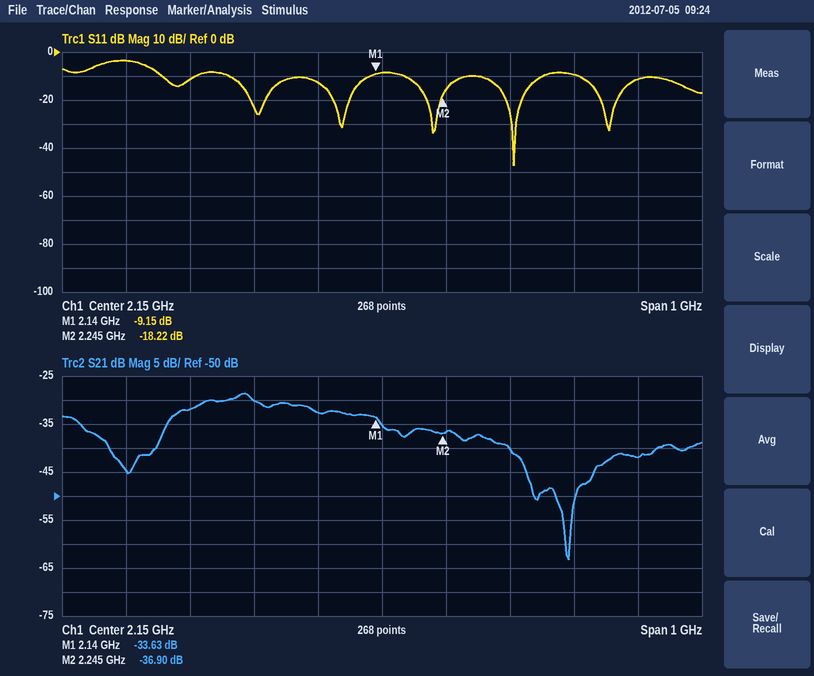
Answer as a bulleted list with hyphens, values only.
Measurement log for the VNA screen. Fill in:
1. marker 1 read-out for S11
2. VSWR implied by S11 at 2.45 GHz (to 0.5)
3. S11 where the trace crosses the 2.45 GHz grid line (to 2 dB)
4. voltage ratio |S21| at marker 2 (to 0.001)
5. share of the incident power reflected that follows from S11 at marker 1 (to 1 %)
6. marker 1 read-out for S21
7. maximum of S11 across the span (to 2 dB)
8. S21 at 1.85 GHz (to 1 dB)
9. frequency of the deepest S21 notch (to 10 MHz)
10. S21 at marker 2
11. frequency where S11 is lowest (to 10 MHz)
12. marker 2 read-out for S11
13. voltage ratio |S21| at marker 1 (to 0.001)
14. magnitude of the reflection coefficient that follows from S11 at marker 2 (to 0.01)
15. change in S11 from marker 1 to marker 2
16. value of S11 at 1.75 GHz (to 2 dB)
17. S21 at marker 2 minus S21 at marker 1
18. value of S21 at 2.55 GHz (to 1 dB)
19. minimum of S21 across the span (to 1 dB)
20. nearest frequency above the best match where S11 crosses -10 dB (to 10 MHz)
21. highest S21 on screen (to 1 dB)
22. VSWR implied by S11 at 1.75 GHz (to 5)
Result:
- -9.15 dB
- 2.0
- -10 dB
- 0.014
- 12 %
- -33.63 dB
- -4 dB
- -32 dB
- 2.44 GHz
- -36.90 dB
- 2.36 GHz
- -18.22 dB
- 0.021
- 0.12
- -9.07 dB
- -4 dB
- -3.27 dB
- -42 dB
- -63 dB
- 2.40 GHz
- -29 dB
- 5
